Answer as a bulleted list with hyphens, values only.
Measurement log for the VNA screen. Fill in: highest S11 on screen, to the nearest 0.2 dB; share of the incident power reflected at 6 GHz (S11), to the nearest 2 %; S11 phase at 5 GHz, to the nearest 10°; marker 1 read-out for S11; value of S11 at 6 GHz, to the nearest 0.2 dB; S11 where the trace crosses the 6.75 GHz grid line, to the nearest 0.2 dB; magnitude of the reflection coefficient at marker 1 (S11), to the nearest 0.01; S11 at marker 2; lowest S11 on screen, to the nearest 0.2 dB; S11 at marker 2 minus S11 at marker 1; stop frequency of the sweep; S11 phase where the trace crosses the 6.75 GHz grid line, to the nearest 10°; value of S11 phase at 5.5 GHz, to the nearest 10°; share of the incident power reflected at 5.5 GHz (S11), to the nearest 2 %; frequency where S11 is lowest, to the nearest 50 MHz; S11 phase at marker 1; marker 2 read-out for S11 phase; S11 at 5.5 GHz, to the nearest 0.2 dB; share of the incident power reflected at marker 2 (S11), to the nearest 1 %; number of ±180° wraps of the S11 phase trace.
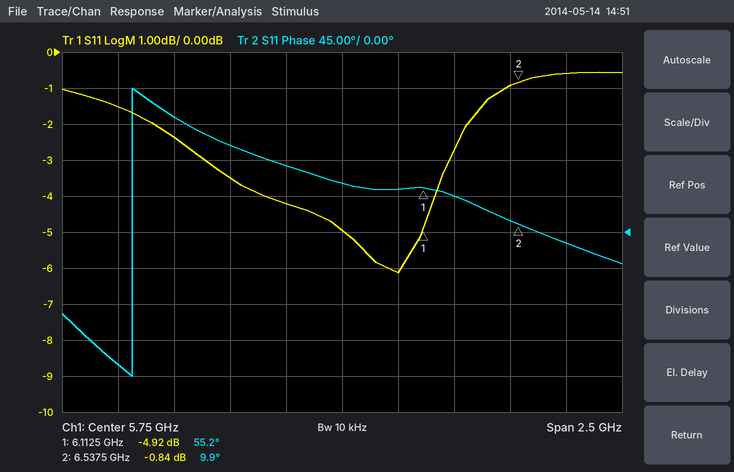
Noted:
- -0.6 dB
- 24 %
- 140°
- -4.92 dB
- -6.2 dB
- -0.6 dB
- 0.57
- -0.84 dB
- -6.2 dB
- 4.08 dB
- 7 GHz
- -10°
- 80°
- 38 %
- 6.00 GHz
- 55.2°
- 9.9°
- -4.2 dB
- 82 %
- 1
